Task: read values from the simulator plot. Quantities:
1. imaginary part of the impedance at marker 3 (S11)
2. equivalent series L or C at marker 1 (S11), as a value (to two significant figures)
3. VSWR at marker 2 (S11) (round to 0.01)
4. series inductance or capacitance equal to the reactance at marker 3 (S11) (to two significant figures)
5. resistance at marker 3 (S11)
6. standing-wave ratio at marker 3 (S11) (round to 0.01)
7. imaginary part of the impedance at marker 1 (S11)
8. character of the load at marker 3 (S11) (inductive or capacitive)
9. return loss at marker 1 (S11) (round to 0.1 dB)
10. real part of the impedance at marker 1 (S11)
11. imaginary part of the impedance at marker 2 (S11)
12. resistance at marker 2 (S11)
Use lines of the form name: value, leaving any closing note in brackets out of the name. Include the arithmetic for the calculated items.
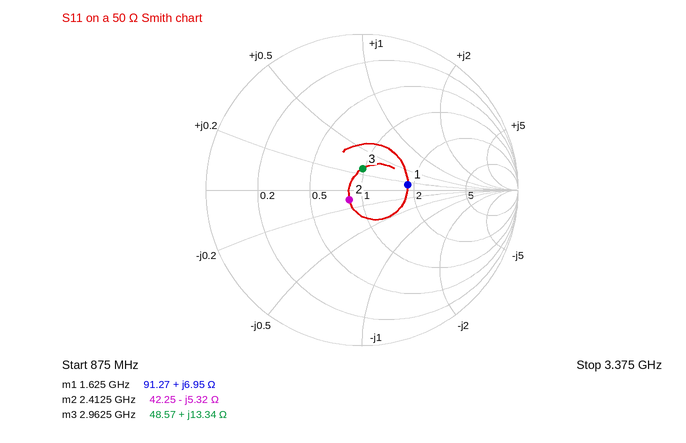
imaginary part of the impedance at marker 3: +13.34 Ω
equivalent series L or C at marker 1 (S11), as a value: L = 6.95 Ω/(2π × 1.625 GHz) ≈ 681 pH, so 680 pH to two significant figures
VSWR at marker 2 (S11): 1.23
series inductance or capacitance equal to the reactance at marker 3 (S11): L = 13.34 Ω/(2π × 2.9625 GHz) ≈ 717 pH, so 720 pH to two significant figures
resistance at marker 3: 48.57 Ω
standing-wave ratio at marker 3 (S11): 1.31
imaginary part of the impedance at marker 1: +6.95 Ω
character of the load at marker 3 (S11): inductive
return loss at marker 1 (S11): 10.6 dB
real part of the impedance at marker 1: 91.27 Ω
imaginary part of the impedance at marker 2: -5.32 Ω
resistance at marker 2: 42.25 Ω
